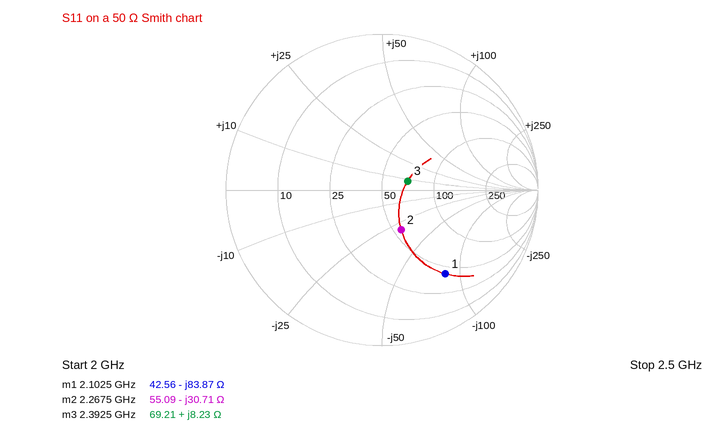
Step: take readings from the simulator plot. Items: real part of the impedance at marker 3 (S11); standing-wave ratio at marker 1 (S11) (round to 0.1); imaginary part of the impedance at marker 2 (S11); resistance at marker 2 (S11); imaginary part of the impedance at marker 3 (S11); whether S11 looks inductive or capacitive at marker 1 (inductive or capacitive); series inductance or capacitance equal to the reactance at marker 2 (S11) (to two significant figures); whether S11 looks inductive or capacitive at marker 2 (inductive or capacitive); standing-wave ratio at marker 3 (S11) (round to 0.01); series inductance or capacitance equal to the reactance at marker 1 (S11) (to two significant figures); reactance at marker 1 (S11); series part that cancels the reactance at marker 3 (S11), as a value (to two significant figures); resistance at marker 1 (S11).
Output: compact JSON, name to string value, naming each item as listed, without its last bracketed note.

{"real part of the impedance at marker 3": "69.21 Ω", "standing-wave ratio at marker 1 (S11)": "5.1", "imaginary part of the impedance at marker 2": "-30.71 Ω", "resistance at marker 2": "55.09 Ω", "imaginary part of the impedance at marker 3": "+8.23 Ω", "whether S11 looks inductive or capacitive at marker 1": "capacitive", "series inductance or capacitance equal to the reactance at marker 2 (S11)": "2.3 pF", "whether S11 looks inductive or capacitive at marker 2": "capacitive", "standing-wave ratio at marker 3 (S11)": "1.42", "series inductance or capacitance equal to the reactance at marker 1 (S11)": "900 fF", "reactance at marker 1": "-83.87 Ω", "series part that cancels the reactance at marker 3 (S11), as a value": "8.1 pF", "resistance at marker 1": "42.56 Ω"}
